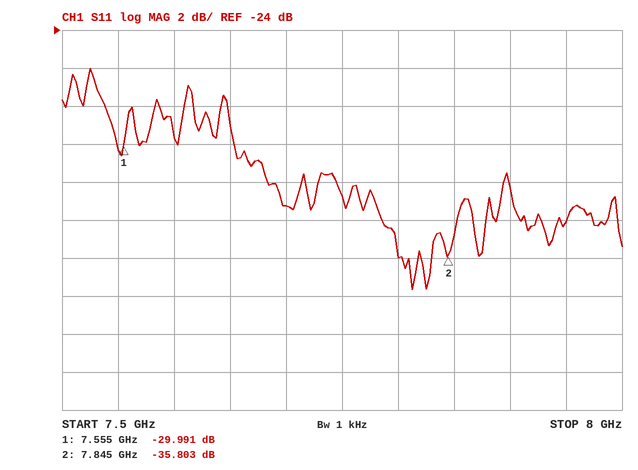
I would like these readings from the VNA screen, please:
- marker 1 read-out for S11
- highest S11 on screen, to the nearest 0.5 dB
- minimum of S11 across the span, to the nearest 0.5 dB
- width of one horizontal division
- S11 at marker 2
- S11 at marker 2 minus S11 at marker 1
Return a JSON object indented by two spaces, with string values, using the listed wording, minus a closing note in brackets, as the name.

{
  "marker 1 read-out for S11": "-29.991 dB",
  "highest S11 on screen, to the nearest 0.5 dB": "-26.0 dB",
  "minimum of S11 across the span, to the nearest 0.5 dB": "-37.5 dB",
  "width of one horizontal division": "50 MHz",
  "S11 at marker 2": "-35.803 dB",
  "S11 at marker 2 minus S11 at marker 1": "-5.812 dB"
}
